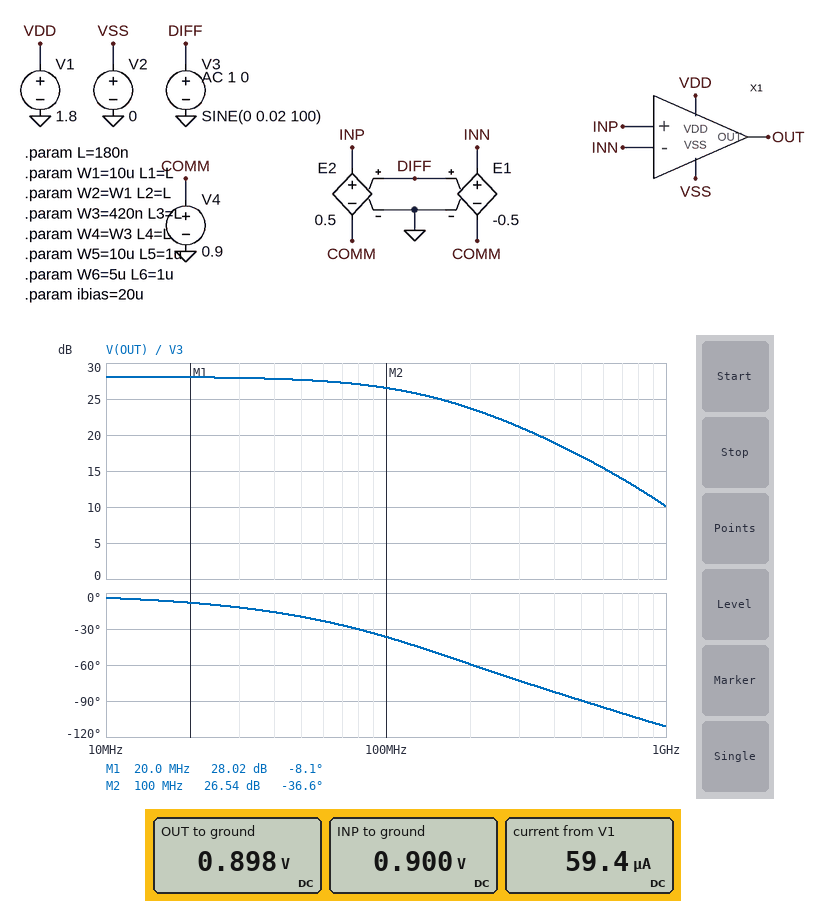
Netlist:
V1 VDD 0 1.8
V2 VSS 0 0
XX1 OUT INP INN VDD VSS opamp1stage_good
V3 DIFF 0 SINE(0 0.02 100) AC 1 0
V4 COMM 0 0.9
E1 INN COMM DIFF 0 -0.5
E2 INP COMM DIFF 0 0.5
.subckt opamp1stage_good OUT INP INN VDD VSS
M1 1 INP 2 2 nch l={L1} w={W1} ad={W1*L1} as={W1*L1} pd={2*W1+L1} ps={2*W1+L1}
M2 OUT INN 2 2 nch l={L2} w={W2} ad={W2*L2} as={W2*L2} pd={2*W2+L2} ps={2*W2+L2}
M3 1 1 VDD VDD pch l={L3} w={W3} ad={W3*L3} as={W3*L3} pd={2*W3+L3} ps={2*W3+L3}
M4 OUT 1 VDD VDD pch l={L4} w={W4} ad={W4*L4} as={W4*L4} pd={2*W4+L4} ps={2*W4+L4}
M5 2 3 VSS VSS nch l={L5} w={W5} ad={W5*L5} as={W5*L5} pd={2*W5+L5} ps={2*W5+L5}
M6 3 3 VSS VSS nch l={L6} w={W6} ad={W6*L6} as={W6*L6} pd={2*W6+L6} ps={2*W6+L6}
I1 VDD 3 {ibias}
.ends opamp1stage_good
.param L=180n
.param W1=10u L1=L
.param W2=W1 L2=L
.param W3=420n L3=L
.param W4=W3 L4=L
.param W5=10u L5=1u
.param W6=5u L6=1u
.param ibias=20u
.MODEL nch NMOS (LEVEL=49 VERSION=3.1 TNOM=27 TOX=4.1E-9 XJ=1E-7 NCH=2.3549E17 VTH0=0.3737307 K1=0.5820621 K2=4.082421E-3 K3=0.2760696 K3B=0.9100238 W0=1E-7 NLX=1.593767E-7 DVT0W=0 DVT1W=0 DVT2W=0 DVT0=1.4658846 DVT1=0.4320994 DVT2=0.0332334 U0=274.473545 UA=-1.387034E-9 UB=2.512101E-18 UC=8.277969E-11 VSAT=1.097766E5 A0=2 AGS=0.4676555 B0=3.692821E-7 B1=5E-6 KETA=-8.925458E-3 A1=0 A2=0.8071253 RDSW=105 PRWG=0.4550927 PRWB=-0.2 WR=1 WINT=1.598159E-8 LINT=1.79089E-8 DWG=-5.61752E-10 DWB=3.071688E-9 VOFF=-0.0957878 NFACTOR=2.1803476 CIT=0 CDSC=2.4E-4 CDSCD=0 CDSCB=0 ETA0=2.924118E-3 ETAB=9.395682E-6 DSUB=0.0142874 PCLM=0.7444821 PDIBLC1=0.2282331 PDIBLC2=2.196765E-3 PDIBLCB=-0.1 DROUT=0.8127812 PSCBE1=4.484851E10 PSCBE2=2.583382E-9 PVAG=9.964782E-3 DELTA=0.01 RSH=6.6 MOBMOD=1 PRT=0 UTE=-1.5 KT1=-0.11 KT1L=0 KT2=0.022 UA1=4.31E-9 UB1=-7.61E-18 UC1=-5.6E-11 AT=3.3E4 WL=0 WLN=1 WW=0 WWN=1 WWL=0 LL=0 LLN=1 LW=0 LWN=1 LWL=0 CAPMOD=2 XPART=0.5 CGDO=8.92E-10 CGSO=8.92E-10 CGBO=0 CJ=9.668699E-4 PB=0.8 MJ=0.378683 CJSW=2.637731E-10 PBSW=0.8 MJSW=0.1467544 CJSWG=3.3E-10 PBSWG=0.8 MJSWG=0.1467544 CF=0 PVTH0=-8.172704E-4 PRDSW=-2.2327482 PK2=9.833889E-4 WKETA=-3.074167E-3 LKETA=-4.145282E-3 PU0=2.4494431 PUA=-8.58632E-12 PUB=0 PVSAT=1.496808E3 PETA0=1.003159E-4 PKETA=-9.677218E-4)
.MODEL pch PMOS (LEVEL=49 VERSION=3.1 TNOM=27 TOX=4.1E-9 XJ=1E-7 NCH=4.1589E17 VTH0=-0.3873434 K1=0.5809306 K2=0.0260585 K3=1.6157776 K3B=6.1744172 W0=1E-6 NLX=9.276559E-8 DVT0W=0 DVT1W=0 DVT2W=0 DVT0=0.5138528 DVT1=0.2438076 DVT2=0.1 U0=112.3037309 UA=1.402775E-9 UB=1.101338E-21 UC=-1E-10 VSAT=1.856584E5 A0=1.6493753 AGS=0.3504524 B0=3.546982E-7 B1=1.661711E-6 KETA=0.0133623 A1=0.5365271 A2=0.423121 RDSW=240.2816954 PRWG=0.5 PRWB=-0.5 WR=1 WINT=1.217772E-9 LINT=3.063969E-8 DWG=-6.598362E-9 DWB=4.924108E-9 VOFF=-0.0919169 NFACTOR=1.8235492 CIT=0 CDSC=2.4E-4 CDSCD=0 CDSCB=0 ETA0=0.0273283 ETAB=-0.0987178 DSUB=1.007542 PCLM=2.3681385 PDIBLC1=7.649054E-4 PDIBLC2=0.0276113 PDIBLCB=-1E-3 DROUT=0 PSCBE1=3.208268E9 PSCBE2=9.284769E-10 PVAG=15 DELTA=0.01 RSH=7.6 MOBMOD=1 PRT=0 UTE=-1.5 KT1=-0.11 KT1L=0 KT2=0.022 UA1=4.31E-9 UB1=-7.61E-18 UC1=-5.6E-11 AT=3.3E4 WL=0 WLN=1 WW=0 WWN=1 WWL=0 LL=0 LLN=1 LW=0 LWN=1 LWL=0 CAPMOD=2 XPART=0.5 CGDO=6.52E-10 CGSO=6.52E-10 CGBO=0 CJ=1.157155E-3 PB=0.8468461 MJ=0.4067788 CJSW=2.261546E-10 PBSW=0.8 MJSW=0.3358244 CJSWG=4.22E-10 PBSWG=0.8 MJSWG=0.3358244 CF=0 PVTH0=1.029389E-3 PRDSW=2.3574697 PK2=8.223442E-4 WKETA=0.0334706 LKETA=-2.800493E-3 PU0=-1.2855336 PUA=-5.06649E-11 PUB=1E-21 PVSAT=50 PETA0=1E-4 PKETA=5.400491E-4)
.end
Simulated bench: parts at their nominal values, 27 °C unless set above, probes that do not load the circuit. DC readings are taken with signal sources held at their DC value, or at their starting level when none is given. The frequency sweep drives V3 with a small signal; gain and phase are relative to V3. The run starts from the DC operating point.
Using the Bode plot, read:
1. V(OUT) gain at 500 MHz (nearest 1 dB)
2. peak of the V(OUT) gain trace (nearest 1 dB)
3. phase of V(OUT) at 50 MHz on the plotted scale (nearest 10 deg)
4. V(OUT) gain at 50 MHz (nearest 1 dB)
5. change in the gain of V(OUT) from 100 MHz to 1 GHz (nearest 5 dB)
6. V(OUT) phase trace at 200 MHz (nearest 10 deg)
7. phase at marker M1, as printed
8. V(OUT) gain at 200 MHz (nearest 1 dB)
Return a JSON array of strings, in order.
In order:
["17 dB", "28 dB", "-20 deg", "28 dB", "-15 dB", "-60 deg", "-8.1 deg", "24 dB"]
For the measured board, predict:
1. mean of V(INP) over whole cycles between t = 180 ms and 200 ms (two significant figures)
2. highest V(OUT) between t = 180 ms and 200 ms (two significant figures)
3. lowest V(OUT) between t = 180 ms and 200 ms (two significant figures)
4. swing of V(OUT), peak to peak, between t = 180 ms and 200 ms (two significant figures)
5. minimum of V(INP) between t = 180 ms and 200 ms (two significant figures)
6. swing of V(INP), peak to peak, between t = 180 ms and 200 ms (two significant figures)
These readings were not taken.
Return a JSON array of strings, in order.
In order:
["900 mV", "1.4 V", "490 mV", "890 mV", "890 mV", "20 mV"]
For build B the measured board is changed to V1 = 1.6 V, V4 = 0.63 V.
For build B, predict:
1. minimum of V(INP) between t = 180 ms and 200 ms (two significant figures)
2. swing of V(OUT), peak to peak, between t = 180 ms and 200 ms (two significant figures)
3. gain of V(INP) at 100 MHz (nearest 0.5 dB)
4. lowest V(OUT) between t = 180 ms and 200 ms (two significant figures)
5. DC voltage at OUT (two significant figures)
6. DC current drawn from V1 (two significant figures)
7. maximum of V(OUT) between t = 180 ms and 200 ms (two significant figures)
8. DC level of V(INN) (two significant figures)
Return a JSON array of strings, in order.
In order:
["620 mV", "940 mV", "-6.0 dB", "260 mV", "720 mV", "56 µA", "1.2 V", "630 mV"]
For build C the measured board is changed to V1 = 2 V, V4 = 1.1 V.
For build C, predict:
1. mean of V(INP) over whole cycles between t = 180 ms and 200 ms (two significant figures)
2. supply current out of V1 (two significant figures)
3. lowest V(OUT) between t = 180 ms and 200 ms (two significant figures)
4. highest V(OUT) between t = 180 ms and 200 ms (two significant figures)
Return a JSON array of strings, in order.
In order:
["1.1 V", "60 µA", "690 mV", "1.6 V"]
